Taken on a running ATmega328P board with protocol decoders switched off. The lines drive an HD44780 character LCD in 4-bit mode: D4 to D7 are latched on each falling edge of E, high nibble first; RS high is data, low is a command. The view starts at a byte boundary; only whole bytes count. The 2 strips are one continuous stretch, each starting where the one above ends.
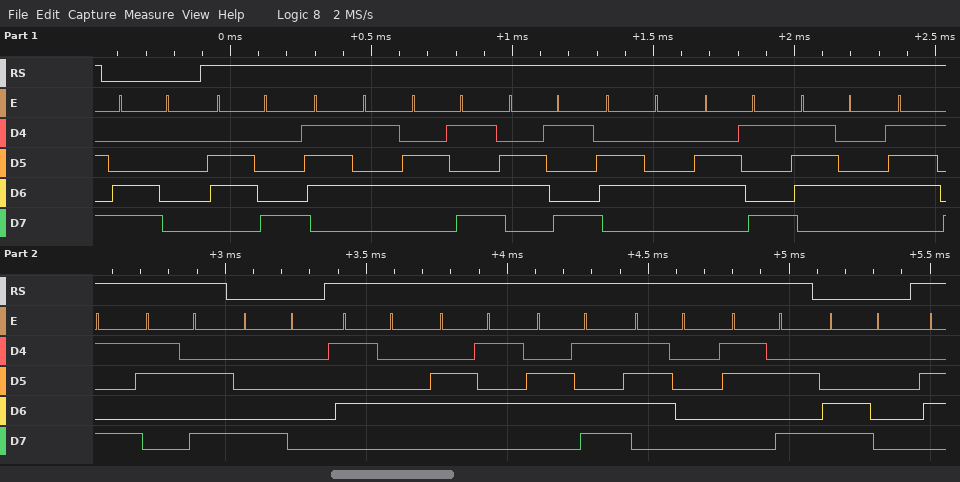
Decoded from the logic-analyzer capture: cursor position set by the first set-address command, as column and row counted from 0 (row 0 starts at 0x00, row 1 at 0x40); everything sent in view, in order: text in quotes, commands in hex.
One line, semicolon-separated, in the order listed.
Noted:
column 0, row 1; 0xC0 "humidity:" 0x80 "Temp:" 0xC0
